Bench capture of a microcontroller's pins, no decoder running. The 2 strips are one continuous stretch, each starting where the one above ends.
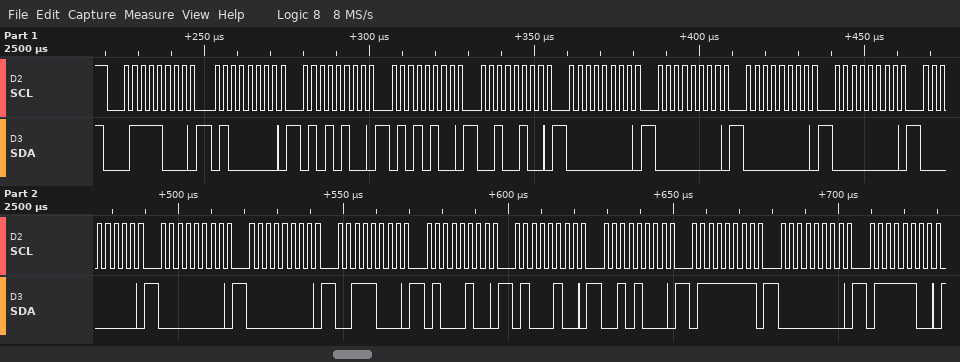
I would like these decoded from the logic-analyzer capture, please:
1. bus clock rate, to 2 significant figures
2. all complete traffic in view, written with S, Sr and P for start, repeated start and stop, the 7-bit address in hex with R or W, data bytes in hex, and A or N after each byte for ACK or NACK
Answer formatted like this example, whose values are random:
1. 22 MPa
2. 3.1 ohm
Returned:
1. 400 kHz
2. S 3CW A 40 A 54 A 54 A 24 A 00 A 00 A 00 A 00 A 00 A 00 A 00 A 38 A 44 A 44 A 28 A 7F A 00 A 7C A
